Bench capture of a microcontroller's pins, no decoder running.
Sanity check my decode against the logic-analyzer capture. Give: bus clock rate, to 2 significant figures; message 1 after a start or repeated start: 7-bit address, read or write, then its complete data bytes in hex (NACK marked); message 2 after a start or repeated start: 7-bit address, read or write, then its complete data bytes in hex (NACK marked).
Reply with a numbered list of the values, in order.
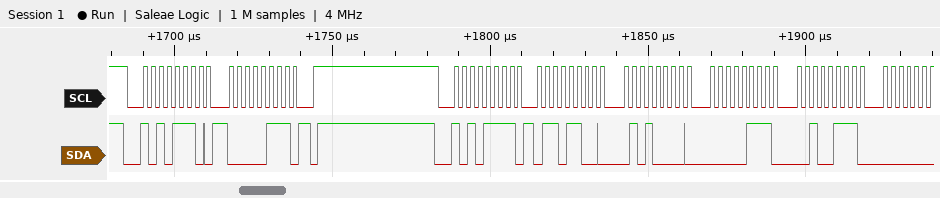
1. 400 kHz
2. 0x57 write: 07
3. 0x57 read: 6C 50 07 27
